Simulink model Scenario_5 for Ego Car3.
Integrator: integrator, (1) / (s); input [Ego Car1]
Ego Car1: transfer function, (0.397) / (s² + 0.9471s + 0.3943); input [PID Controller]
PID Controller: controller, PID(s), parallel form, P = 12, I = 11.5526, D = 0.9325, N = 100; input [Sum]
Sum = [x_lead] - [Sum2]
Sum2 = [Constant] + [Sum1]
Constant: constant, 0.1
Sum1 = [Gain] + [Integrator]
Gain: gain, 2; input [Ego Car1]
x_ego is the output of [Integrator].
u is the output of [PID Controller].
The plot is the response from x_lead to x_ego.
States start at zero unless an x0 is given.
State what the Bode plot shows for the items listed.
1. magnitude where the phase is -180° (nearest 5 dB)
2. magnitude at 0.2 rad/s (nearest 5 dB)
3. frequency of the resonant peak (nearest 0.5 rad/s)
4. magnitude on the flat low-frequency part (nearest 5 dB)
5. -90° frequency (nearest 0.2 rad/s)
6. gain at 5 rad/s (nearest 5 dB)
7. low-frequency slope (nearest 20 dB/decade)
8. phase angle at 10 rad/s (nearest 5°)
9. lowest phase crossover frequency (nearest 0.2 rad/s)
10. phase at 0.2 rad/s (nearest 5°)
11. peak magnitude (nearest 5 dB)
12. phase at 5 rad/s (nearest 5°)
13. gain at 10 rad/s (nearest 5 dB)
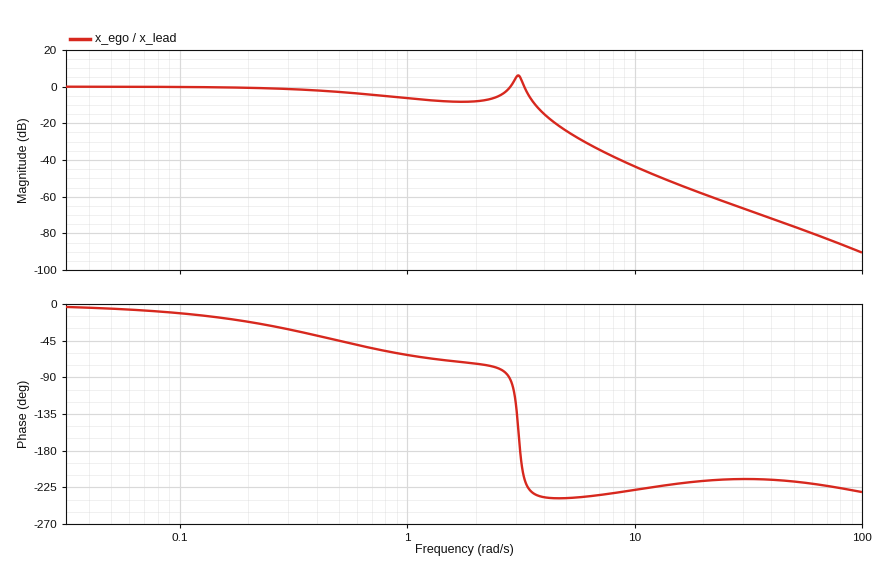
5 dB
0 dB
3.0 rad/s
0 dB
2.8 rad/s
-25 dB
0 dB/decade
-230°
3.2 rad/s
-20°
5 dB
-240°
-45 dB
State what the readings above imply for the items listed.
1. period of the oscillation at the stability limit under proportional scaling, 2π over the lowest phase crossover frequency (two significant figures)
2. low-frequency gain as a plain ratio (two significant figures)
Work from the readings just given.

2.0 s
1.0
